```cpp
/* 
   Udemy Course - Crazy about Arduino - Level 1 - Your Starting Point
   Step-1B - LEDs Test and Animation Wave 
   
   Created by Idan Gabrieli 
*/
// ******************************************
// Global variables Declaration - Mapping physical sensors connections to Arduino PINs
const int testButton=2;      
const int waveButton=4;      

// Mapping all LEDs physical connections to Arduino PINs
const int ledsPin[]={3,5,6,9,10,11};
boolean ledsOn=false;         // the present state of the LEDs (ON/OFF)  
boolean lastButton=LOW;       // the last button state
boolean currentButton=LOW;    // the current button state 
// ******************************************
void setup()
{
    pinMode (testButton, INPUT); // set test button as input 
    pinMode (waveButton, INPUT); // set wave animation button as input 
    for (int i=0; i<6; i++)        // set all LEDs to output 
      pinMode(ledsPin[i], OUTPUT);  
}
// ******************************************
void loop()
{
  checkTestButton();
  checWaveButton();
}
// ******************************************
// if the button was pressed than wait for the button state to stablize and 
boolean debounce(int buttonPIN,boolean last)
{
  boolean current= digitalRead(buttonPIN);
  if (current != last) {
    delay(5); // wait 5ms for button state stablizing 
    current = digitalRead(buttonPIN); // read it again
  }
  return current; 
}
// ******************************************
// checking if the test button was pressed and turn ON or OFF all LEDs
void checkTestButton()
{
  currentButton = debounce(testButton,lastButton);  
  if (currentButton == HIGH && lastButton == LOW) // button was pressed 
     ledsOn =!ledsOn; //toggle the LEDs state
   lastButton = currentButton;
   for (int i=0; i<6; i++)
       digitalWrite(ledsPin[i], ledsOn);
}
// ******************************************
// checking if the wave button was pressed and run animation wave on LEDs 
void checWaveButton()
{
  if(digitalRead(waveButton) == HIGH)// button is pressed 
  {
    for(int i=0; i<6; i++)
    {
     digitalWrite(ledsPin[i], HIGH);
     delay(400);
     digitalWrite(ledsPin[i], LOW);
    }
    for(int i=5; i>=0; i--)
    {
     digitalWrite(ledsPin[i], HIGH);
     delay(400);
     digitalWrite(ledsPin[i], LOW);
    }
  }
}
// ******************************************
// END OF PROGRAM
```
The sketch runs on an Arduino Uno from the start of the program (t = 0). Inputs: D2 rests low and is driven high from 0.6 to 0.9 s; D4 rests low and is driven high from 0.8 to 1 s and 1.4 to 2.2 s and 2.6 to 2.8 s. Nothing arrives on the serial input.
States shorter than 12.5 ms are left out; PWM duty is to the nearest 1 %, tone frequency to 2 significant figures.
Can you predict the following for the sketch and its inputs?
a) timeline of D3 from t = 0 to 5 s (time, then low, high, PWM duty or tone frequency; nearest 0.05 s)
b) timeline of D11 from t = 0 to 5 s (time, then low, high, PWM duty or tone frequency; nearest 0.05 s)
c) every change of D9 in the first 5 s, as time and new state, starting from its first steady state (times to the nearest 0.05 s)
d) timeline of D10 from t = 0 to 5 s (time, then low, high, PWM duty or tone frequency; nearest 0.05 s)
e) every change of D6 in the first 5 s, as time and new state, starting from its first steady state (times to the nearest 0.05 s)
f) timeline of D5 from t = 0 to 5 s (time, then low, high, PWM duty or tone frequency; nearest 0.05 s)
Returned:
0 s low; 0.6 s high; 1.2 s low
0 s low; 0.6 s high; 3.6 s low
0 s low; 0.6 s high; 2.4 s low; 4 s high; 4.4 s low
0 s low; 0.6 s high; 2.8 s low; 3.6 s high; 4 s low
0 s low; 0.6 s high; 2 s low; 4.4 s high; 4.8 s low
0 s low; 0.6 s high; 1.6 s low; 4.8 s high
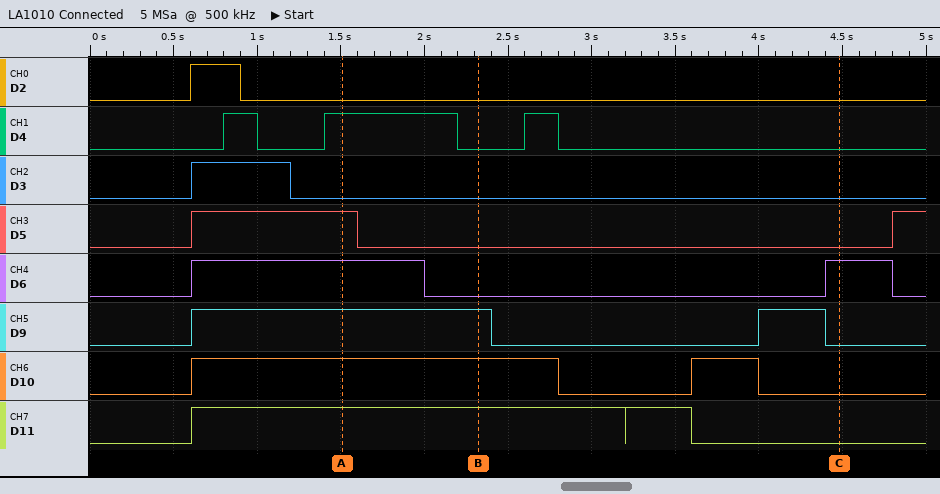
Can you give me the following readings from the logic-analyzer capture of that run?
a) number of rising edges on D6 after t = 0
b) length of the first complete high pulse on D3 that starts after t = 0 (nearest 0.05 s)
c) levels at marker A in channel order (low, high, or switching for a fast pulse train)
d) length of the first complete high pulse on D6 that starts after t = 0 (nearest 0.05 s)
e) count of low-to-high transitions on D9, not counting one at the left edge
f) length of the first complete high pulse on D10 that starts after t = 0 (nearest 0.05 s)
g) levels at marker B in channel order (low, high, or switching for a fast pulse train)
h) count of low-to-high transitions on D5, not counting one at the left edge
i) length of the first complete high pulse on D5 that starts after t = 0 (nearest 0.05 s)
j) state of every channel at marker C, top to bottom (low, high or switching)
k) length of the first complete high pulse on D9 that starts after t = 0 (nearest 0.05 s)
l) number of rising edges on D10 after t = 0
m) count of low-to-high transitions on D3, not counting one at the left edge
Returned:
2
0.60 s
D2 low, D4 high, D3 low, D5 high, D6 high, D9 high, D10 high, D11 high
1.40 s
2
2.20 s
D2 low, D4 low, D3 low, D5 low, D6 low, D9 high, D10 high, D11 high
2
1.00 s
D2 low, D4 low, D3 low, D5 low, D6 high, D9 low, D10 low, D11 low
1.80 s
2
1
